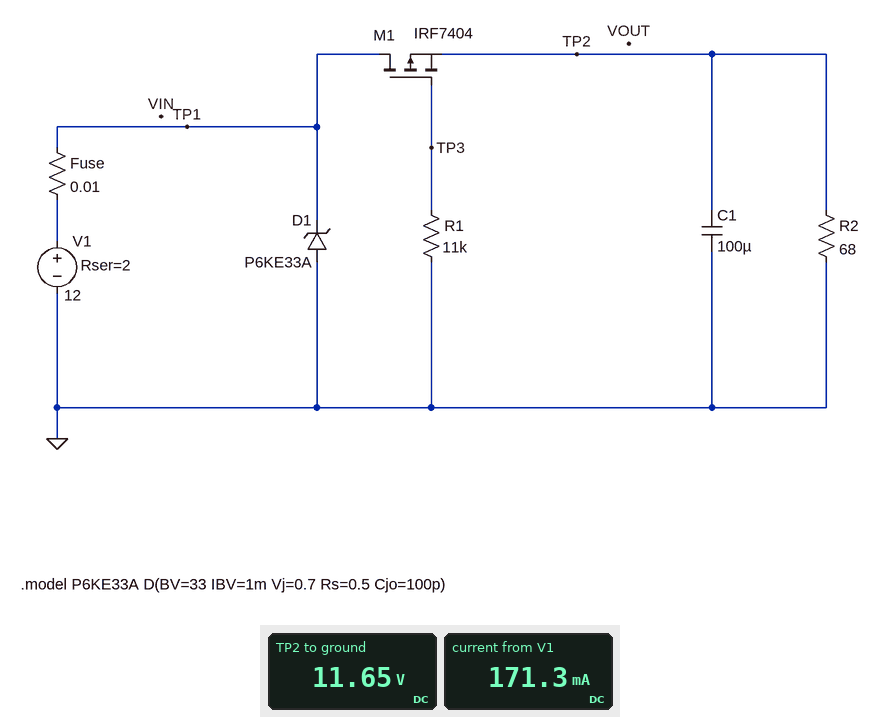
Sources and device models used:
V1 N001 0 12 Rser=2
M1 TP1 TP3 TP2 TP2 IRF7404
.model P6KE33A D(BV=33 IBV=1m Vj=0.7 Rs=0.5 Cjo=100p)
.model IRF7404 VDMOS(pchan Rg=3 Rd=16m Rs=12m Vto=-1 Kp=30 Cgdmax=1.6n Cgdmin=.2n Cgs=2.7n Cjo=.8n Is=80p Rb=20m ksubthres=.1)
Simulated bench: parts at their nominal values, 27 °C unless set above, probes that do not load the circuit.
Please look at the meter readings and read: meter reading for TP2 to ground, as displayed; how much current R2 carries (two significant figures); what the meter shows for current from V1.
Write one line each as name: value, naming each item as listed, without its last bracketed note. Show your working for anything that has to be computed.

meter reading for TP2 to ground, as displayed: 11.65 V
how much current R2 carries: (11.65 V) / 68 Ω = 170 mA
what the meter shows for current from V1: 171.3 mA
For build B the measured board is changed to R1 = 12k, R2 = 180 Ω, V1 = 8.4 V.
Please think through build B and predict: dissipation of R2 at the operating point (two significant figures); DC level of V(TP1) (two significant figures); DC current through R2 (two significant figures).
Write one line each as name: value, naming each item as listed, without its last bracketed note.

dissipation of R2 at the operating point: 380 mW
DC level of V(TP1): 8.3 V
DC current through R2: 46 mA
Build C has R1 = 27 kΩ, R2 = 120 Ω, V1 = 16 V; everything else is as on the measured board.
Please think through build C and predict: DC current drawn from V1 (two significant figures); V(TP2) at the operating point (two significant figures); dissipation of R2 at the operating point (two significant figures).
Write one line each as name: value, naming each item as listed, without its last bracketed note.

DC current drawn from V1: 130 mA
V(TP2) at the operating point: 16 V
dissipation of R2 at the operating point: 2.1 W
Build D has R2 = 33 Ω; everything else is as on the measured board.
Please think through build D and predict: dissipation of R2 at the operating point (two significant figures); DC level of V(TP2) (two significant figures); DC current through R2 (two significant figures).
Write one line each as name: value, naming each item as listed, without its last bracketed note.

dissipation of R2 at the operating point: 3.9 W
DC level of V(TP2): 11 V
DC current through R2: 340 mA
